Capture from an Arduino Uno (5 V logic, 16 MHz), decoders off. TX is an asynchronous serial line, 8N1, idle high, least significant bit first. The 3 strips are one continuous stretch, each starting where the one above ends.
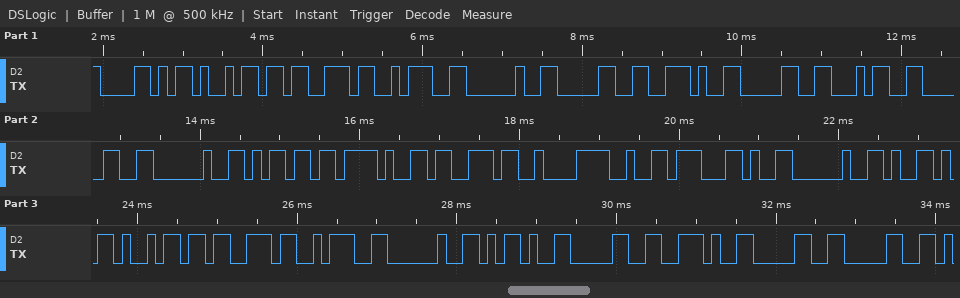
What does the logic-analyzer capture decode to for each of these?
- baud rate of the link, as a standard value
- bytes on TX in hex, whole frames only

9600 baud
58 69 73 3A 20 30 2E 30 34 30 20 6D 2F 73 C2 B2 2C 20 59 69 73 3A 20 2D 30 2E 30 30
